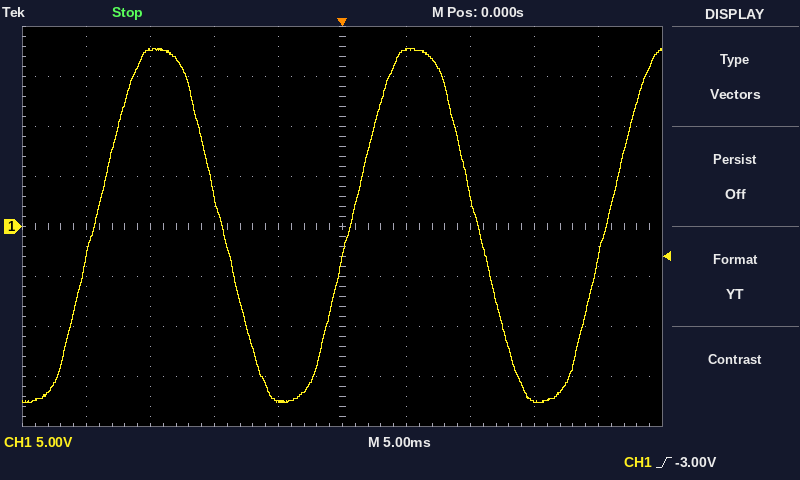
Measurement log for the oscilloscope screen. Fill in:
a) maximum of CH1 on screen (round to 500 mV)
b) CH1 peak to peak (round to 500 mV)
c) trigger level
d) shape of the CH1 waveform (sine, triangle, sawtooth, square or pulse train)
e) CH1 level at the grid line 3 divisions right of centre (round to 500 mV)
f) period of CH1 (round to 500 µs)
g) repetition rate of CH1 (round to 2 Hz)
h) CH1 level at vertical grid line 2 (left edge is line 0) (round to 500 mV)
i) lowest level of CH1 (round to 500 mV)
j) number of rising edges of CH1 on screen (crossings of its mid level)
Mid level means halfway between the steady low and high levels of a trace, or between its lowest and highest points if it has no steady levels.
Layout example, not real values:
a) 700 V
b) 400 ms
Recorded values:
a) 18.0 V
b) 35.5 V
c) -3.00 V
d) sine
e) -17.5 V
f) 20.0 ms
g) 50 Hz
h) 17.5 V
i) -17.5 V
j) 3
